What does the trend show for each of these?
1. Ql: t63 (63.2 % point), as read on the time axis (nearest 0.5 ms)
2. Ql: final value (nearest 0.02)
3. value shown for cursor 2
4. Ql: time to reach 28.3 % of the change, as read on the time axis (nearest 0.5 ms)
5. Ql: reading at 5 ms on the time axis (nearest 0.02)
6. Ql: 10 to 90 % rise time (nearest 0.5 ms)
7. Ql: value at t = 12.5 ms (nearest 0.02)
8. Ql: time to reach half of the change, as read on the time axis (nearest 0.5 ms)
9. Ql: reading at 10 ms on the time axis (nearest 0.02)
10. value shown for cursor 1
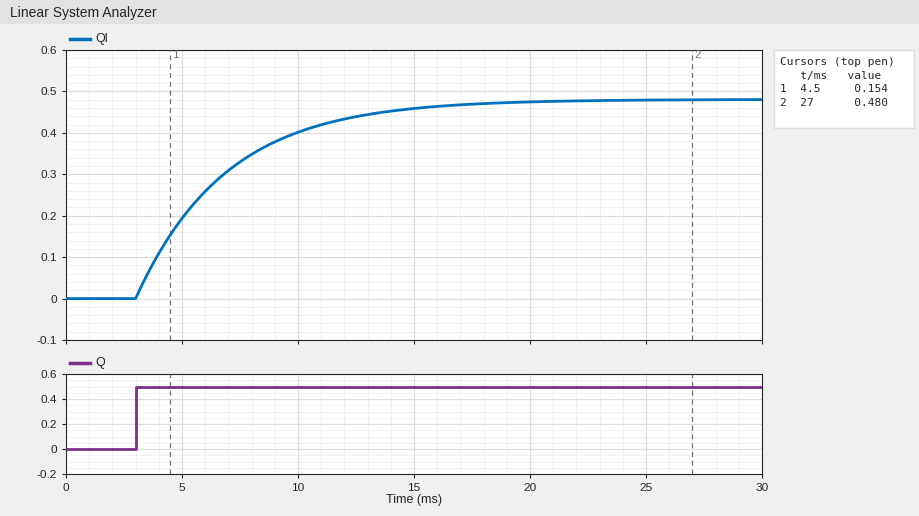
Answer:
7.0 ms
0.48
0.480
4.5 ms
0.20
8.5 ms
0.44
5.5 ms
0.40
0.154
